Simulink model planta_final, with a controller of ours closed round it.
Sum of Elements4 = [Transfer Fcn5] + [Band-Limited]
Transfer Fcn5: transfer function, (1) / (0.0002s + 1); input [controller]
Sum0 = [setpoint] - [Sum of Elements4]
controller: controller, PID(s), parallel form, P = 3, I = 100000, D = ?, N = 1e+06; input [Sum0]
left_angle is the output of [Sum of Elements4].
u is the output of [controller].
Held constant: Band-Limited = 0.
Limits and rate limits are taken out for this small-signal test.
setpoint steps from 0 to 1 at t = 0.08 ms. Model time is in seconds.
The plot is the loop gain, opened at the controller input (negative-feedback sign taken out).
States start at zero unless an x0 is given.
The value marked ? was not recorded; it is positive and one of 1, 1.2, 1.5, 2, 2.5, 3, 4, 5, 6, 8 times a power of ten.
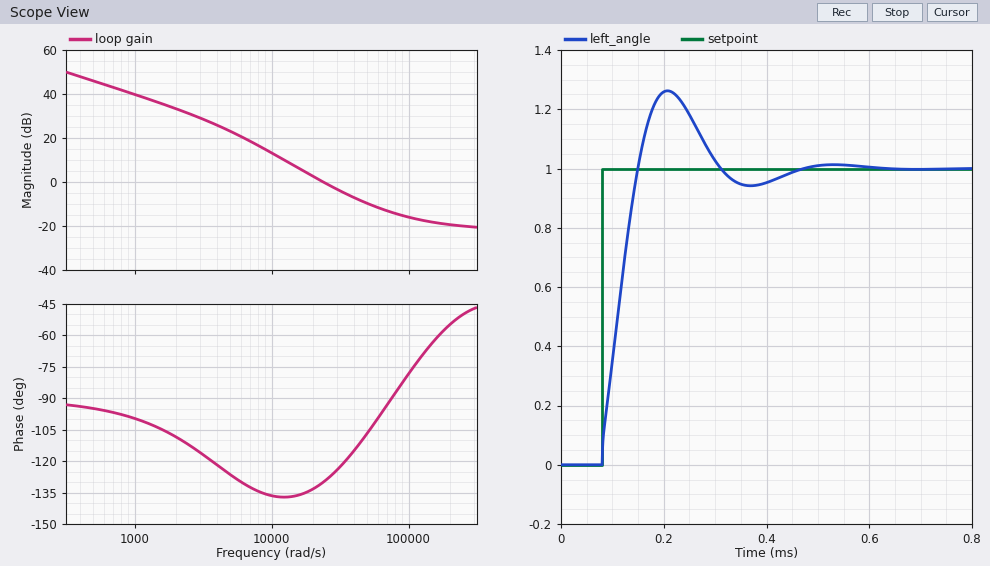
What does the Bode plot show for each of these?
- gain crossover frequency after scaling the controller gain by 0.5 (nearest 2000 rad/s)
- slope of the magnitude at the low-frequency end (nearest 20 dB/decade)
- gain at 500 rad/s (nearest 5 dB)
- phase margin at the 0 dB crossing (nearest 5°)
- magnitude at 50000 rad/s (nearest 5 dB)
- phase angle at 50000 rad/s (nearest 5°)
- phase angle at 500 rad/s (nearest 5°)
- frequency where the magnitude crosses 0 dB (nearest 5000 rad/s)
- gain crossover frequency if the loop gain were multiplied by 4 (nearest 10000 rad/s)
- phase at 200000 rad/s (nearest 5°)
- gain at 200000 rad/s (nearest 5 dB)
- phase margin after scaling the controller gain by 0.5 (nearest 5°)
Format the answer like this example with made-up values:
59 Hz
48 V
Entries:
16000 rad/s
-20 dB/decade
45 dB
50°
-10 dB
-105°
-95°
25000 rad/s
60000 rad/s
-55°
-20 dB
45°
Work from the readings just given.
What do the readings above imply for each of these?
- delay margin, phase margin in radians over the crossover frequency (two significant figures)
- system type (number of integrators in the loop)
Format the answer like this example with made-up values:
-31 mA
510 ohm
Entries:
0.000035 s
1
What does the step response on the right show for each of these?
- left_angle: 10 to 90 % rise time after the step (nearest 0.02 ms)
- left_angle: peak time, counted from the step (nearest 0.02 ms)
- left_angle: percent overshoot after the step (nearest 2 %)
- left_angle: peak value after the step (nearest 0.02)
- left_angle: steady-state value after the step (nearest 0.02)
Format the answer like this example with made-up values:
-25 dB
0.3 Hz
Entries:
0.06 ms
0.12 ms
26 %
1.26
1.00
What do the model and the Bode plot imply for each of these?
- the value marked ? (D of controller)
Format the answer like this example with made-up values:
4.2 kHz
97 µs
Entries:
1.5e-05
